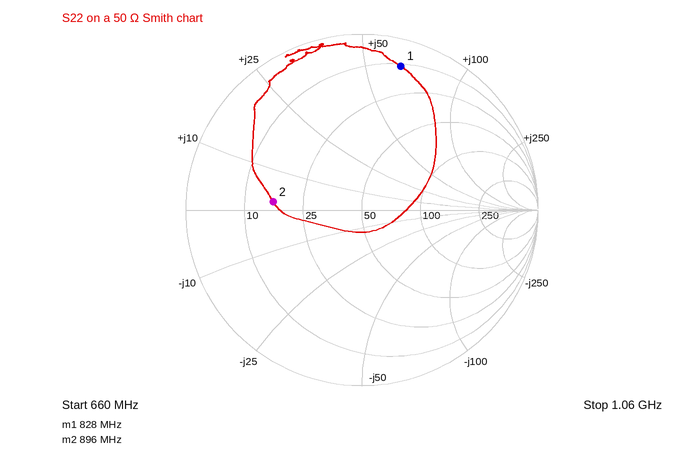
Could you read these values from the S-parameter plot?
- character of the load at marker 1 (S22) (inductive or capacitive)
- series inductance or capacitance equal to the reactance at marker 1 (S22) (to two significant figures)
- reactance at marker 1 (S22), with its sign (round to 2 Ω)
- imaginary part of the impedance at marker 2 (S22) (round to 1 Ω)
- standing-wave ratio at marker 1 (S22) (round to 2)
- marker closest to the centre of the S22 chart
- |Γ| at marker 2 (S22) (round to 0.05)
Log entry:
inductive
12 nH
+64 Ω
+2 Ω
12
marker 2
0.50
